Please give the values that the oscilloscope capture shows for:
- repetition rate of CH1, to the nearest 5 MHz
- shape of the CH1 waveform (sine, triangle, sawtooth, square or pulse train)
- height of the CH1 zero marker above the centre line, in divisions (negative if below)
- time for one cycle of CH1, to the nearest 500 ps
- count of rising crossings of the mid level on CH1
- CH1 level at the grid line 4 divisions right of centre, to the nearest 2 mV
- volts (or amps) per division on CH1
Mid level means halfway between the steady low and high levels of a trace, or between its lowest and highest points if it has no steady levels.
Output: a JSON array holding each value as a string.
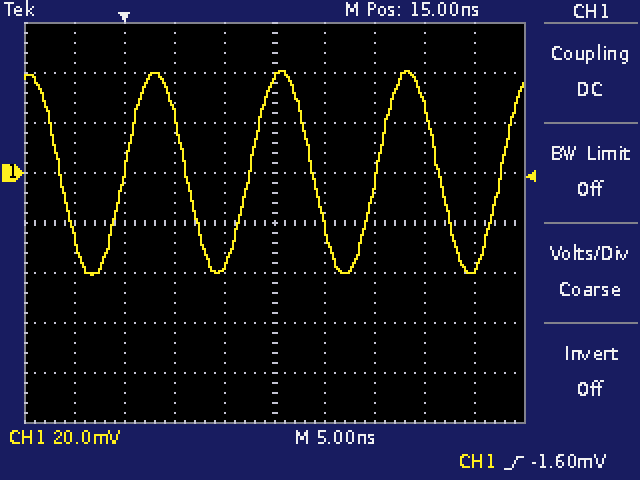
["80 MHz", "sine", "+1.0 div", "12.5 ns", "4", "-38 mV", "20 mV"]
